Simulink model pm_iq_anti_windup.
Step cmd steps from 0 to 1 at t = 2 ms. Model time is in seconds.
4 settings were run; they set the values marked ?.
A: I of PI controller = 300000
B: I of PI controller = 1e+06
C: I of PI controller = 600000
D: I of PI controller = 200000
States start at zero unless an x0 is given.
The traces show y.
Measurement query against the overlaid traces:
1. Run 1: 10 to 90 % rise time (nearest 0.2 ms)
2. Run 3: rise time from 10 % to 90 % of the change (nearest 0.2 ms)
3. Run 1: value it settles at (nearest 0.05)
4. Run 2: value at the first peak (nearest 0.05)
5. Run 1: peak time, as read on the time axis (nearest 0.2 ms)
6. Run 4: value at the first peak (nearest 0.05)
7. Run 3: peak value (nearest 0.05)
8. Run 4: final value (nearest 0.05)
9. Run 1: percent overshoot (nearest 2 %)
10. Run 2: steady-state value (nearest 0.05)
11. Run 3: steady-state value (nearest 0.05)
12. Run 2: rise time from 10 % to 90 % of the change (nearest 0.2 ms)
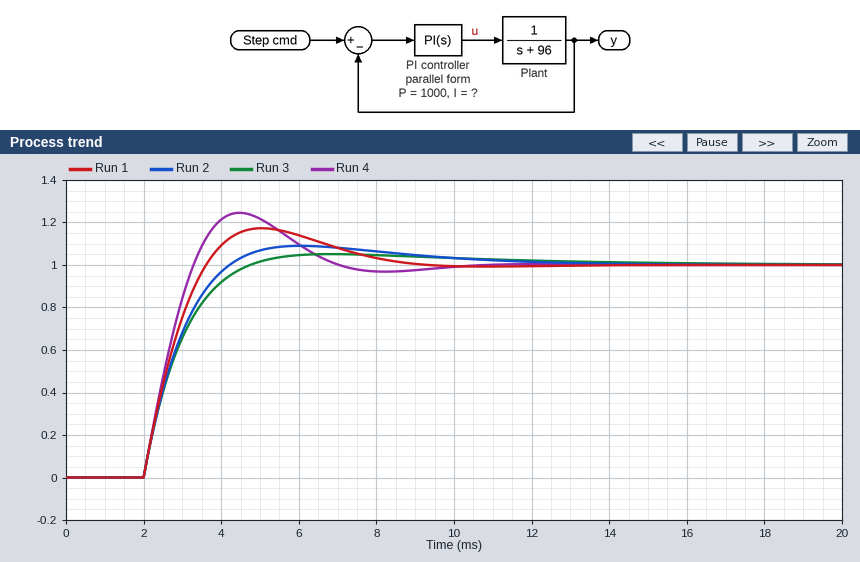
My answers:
1.2 ms
1.8 ms
1.00
1.10
5.0 ms
1.25
1.05
1.00
18 %
1.00
1.00
1.6 ms
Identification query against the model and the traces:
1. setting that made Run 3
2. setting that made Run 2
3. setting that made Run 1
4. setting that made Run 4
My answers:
D
A
C
B
